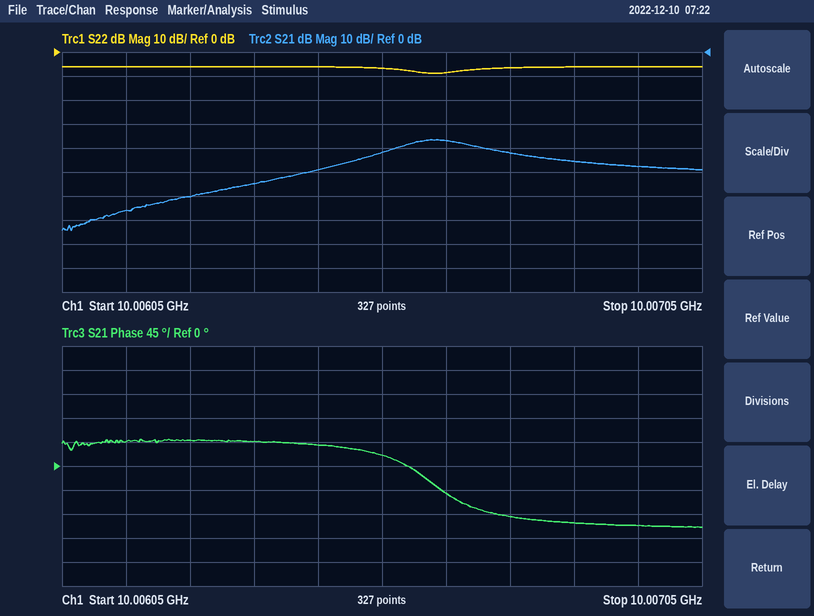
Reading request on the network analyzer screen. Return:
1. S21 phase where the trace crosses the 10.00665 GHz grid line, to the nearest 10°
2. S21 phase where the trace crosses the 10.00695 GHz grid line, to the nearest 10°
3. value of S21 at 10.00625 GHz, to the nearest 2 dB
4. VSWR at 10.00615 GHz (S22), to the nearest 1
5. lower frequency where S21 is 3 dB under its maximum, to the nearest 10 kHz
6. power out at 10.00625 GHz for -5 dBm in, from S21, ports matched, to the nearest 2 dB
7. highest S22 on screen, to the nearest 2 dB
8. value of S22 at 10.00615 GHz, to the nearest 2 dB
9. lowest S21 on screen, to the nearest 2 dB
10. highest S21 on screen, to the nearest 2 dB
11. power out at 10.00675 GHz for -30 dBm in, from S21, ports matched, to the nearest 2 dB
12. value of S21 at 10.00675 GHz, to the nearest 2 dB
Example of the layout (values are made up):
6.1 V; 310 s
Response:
-50°; -110°; -60 dB; 3; 10.00658 GHz; -66 dBm; -6 dB; -6 dB; -74 dB; -36 dB; -72 dBm; -42 dB
